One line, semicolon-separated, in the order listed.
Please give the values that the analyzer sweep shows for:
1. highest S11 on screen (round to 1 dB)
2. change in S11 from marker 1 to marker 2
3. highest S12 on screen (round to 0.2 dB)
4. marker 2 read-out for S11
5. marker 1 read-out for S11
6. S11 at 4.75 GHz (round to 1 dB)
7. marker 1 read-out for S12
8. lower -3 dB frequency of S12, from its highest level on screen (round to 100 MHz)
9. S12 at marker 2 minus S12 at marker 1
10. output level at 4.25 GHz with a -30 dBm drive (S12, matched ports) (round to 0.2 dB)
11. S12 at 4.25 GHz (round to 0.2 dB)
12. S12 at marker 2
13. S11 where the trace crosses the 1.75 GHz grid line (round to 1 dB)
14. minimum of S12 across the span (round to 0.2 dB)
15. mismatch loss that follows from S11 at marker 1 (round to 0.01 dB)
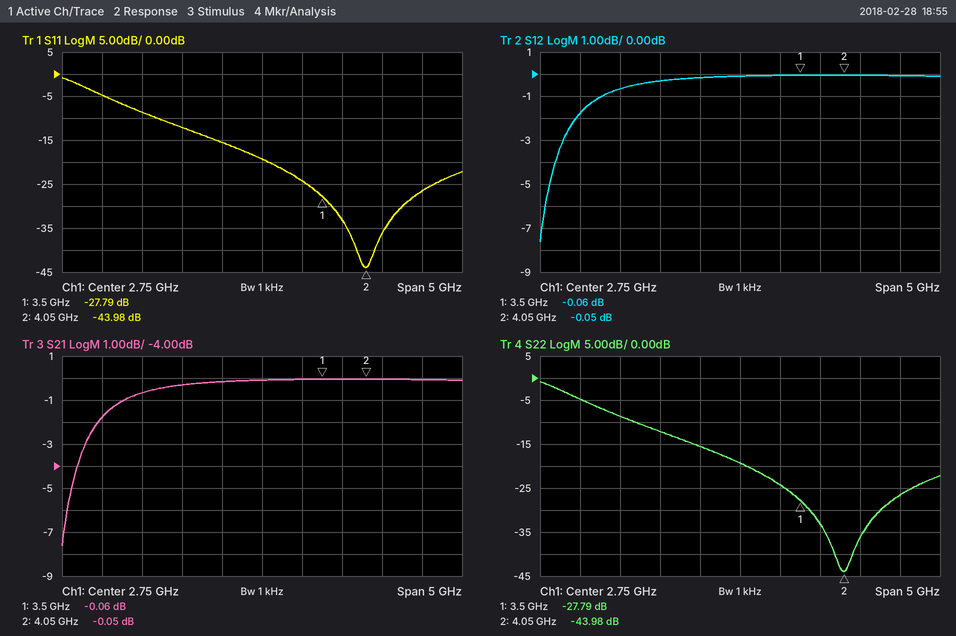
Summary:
-1 dB; -16.19 dB; 0.0 dB; -43.98 dB; -27.79 dB; -27 dB; -0.06 dB; 500 MHz; 0.01 dB; -30.0 dBm; 0.0 dB; -0.05 dB; -12 dB; -7.6 dB; 0.01 dB
